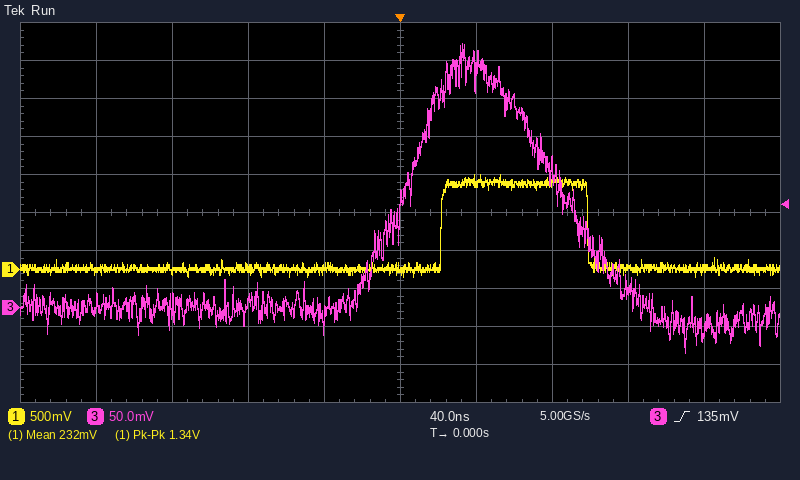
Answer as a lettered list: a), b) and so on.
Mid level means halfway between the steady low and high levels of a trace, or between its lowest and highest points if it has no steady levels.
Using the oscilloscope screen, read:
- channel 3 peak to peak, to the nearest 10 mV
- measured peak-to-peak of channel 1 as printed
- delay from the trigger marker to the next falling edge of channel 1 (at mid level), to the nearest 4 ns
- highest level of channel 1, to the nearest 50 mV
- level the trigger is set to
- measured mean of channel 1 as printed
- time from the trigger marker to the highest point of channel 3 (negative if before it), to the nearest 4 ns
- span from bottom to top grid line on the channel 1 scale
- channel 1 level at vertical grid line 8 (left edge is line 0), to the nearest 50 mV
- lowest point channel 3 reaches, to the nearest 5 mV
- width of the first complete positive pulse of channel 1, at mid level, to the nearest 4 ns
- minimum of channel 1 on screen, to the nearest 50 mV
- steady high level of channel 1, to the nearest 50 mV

a) 410 mV
b) 1.34 V
c) 100 ns
d) 1.25 V
e) 135 mV
f) 232 mV
g) +32 ns
h) 5 V
i) 0 mV
j) -60 mV
k) 76 ns
l) -100 mV
m) 1.15 V
